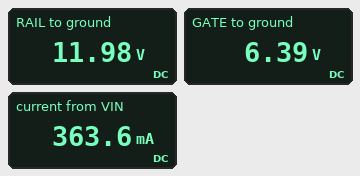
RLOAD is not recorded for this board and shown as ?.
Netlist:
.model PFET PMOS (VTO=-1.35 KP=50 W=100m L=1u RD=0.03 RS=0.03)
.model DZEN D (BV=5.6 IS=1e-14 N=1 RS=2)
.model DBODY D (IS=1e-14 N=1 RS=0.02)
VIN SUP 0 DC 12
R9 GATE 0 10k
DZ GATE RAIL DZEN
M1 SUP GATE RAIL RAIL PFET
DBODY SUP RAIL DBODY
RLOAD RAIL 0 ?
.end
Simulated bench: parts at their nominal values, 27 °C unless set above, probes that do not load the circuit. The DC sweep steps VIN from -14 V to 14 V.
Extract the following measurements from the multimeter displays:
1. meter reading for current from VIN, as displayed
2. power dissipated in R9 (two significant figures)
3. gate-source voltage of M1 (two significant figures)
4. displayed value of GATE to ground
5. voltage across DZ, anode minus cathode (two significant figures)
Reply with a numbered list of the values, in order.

1. 363.6 mA
2. 4.1 mW
3. -5.6 V
4. 6.39 V
5. -5.6 V
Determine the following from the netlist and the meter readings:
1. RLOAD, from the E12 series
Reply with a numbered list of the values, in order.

1. 33 Ω
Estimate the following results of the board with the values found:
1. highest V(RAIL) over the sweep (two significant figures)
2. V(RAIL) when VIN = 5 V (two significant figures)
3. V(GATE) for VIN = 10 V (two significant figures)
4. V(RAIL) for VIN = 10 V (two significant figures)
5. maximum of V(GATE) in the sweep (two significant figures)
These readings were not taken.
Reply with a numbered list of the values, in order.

1. 14 V
2. 5.0 V
3. 4.4 V
4. 10 V
5. 8.4 V
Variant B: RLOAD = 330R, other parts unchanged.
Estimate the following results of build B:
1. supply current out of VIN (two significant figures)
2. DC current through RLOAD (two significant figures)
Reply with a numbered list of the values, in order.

1. 37 mA
2. 36 mA
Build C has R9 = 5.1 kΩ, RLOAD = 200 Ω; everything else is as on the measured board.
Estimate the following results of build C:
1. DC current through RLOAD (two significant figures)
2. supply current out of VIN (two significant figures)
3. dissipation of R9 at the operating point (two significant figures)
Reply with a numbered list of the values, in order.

1. 60 mA
2. 61 mA
3. 8.0 mW
